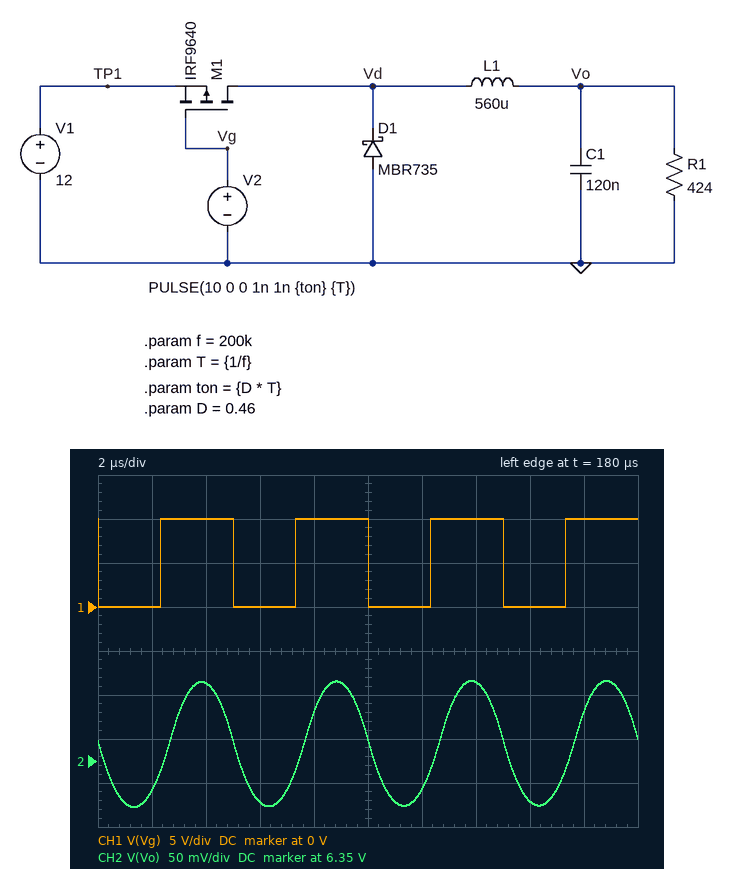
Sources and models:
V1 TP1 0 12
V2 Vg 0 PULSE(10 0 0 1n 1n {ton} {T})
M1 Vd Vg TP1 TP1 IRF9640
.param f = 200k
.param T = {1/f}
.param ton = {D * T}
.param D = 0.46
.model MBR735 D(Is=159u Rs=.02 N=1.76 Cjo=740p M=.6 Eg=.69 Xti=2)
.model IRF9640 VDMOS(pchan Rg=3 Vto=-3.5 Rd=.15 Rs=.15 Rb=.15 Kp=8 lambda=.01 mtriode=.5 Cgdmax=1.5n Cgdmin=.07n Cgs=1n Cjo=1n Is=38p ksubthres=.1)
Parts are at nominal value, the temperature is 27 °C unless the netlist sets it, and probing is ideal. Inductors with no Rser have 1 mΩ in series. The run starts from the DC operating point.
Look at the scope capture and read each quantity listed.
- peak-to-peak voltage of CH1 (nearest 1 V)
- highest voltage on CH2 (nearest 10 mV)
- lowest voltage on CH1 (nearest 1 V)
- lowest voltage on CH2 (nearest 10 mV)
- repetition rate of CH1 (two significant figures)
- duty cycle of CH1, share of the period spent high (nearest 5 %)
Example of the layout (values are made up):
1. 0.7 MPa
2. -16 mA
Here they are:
1. 10 V
2. 6.44 V
3. 0 V
4. 6.30 V
5. 200 kHz
6. 55 %
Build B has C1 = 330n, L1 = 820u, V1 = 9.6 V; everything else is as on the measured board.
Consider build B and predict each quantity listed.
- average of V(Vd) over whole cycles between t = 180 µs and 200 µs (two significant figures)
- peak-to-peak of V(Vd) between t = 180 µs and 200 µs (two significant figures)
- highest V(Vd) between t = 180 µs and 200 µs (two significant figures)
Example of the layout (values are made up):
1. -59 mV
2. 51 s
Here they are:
1. 5.0 V
2. 11 V
3. 10 V
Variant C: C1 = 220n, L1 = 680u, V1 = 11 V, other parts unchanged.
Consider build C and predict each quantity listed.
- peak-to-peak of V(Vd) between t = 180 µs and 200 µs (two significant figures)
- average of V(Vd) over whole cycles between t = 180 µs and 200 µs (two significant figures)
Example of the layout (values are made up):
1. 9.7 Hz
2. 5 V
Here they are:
1. 12 V
2. 5.8 V
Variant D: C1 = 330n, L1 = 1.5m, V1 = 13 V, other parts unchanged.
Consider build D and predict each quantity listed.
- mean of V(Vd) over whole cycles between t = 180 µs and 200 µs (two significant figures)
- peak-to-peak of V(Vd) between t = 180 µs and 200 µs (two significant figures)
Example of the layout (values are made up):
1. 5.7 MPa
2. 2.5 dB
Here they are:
1. 7.3 V
2. 14 V
